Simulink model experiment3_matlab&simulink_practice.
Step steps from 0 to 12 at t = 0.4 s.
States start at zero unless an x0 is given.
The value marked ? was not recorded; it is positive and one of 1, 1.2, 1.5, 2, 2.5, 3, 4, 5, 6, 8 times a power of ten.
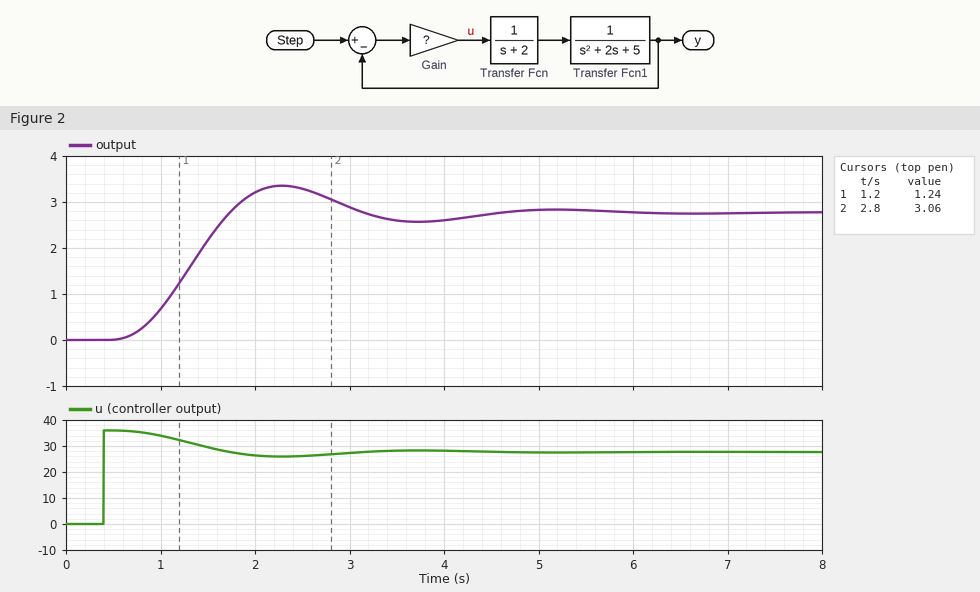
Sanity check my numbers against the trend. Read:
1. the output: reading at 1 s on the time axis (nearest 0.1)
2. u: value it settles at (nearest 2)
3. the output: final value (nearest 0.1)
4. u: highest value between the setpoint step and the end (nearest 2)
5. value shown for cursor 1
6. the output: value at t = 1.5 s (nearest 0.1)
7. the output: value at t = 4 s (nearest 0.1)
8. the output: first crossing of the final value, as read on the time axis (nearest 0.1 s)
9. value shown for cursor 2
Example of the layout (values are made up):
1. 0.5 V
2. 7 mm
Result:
1. 0.7
2. 28
3. 2.8
4. 36
5. 1.24
6. 2.2
7. 2.6
8. 1.7 s
9. 3.06
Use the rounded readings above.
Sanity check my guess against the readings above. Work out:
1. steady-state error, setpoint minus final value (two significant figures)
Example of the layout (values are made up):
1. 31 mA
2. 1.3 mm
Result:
1. 9.2
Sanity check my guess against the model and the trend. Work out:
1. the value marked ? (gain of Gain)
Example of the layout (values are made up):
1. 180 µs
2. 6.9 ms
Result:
1. 3
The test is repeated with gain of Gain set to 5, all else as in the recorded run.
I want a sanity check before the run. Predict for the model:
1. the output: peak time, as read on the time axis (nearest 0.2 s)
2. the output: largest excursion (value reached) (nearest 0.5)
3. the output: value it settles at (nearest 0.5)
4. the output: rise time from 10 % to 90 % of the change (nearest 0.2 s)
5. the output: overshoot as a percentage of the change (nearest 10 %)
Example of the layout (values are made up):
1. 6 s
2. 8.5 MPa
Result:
1. 2.2 s
2. 5.0
3. 4.0
4. 0.8 s
5. 30 %
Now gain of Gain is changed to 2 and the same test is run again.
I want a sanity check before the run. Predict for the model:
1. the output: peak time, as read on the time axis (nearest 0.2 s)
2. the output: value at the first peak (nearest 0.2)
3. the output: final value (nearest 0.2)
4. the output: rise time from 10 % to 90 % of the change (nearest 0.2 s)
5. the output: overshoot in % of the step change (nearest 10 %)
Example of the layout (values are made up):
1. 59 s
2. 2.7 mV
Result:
1. 2.4 s
2. 2.4
3. 2.0
4. 0.8 s
5. 20 %
